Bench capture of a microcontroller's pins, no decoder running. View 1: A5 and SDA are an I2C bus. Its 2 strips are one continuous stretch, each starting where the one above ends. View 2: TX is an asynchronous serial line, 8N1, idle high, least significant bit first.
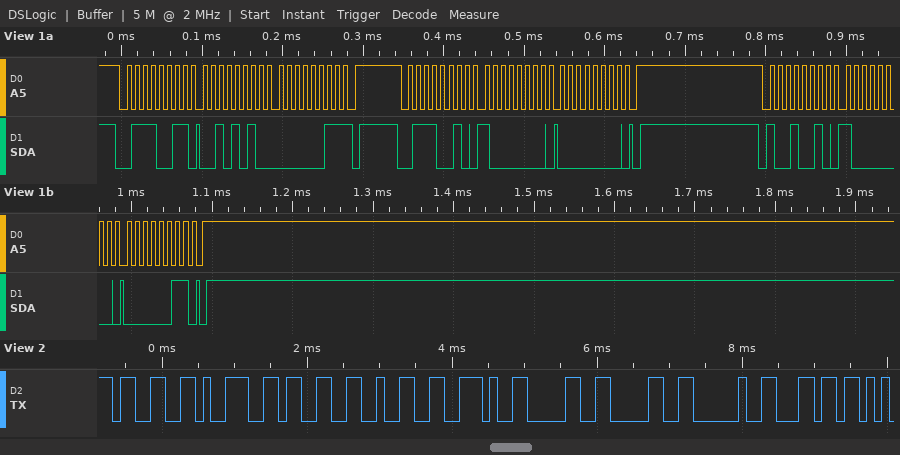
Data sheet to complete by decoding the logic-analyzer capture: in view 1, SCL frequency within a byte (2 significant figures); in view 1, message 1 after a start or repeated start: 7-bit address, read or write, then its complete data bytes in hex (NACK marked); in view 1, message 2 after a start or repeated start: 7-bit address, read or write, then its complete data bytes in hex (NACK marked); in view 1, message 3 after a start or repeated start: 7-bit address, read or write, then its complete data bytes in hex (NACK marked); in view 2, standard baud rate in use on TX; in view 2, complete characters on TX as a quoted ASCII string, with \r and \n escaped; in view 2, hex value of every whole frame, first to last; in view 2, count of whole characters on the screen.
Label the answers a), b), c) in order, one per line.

a) 100 kHz
b) 0x39 read: 2A 03 NACK
c) 0x39 write: 80 00
d) 0x49 write: 80 03
e) 9600 baud
f) "3932.00 l"
g) 33 39 33 32 2E 30 30 20 6C
h) 9
